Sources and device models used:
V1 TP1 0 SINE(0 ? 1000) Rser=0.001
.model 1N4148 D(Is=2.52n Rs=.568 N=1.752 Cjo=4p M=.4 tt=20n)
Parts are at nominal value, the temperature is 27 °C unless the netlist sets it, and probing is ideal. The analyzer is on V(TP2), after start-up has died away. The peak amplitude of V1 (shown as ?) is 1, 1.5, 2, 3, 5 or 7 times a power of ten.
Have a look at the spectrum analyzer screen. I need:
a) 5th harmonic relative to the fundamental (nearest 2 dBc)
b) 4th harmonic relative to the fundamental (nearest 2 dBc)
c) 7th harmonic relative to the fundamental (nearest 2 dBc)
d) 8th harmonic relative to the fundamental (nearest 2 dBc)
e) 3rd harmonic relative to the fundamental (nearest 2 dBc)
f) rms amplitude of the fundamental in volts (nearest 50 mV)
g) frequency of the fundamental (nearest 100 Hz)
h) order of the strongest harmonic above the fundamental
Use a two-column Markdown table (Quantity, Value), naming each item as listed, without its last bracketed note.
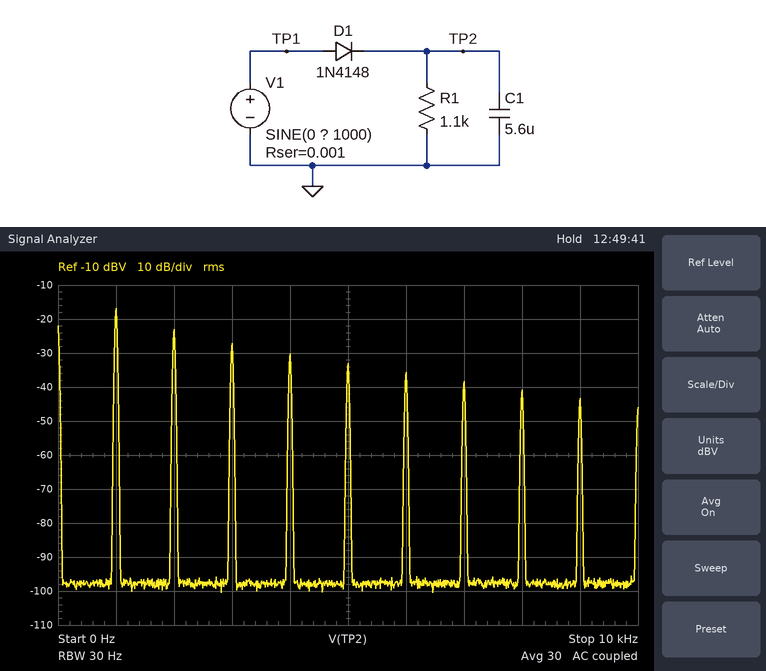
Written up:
| Quantity | Value |
|---|---|
| 5th harmonic relative to the fundamental | -16 dBc |
| 4th harmonic relative to the fundamental | -14 dBc |
| 7th harmonic relative to the fundamental | -22 dBc |
| 8th harmonic relative to the fundamental | -24 dBc |
| 3rd harmonic relative to the fundamental | -10 dBc |
| rms amplitude of the fundamental in volts | 150 mV |
| frequency of the fundamental | 1.0 kHz |
| order of the strongest harmonic above the fundamental | 2 |
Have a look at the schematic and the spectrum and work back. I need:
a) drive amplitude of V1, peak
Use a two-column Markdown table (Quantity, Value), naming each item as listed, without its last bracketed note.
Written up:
| Quantity | Value |
|---|---|
| drive amplitude of V1, peak | 5 V |
